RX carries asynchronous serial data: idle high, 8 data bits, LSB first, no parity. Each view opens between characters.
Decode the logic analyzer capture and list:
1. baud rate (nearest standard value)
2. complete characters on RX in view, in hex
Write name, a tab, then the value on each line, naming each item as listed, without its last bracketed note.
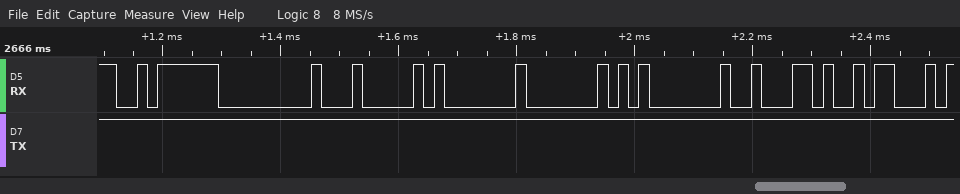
baud rate	57600 baud
complete characters on RX in view, in hex	FA, 00, 04, 01, 40, 01, 62, 1A
